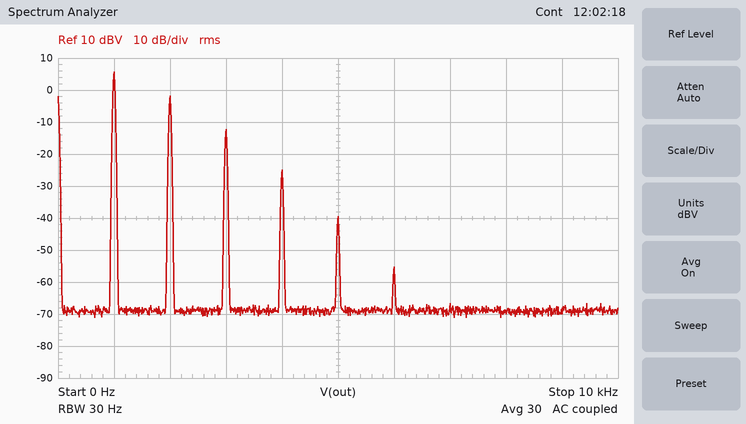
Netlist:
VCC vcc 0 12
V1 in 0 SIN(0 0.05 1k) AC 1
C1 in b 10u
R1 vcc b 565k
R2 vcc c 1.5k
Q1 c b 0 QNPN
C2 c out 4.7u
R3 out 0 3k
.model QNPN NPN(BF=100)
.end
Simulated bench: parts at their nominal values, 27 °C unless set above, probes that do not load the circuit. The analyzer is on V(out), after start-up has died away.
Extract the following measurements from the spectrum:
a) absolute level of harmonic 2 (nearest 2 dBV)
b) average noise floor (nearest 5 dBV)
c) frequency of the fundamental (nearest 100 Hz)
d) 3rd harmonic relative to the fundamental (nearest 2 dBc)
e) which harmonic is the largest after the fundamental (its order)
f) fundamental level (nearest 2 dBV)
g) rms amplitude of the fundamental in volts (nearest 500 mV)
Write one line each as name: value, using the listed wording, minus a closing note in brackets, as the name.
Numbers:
absolute level of harmonic 2: -2 dBV
average noise floor: -70 dBV
frequency of the fundamental: 1.0 kHz
3rd harmonic relative to the fundamental: -18 dBc
which harmonic is the largest after the fundamental: 2
fundamental level: 6 dBV
rms amplitude of the fundamental in volts: 2.0 V
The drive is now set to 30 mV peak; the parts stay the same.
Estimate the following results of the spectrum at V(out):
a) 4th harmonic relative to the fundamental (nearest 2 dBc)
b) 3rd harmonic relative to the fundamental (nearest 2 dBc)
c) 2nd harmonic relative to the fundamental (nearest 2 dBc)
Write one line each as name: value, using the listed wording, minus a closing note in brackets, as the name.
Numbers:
4th harmonic relative to the fundamental: -42 dBc
3rd harmonic relative to the fundamental: -26 dBc
2nd harmonic relative to the fundamental: -12 dBc
